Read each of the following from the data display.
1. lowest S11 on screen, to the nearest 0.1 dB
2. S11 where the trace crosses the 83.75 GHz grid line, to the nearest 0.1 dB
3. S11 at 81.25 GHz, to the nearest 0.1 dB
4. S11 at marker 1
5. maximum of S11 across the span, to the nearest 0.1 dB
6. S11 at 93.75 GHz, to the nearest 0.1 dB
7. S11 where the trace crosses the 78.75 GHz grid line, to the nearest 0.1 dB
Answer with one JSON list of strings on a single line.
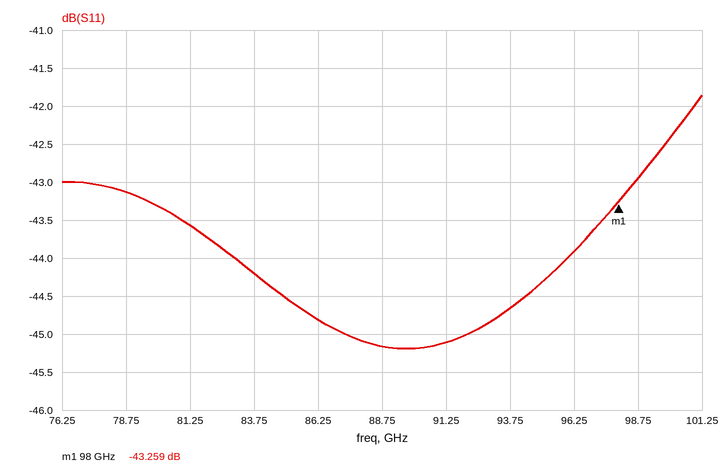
["-45.2 dB", "-44.2 dB", "-43.6 dB", "-43.259 dB", "-41.9 dB", "-44.7 dB", "-43.1 dB"]
